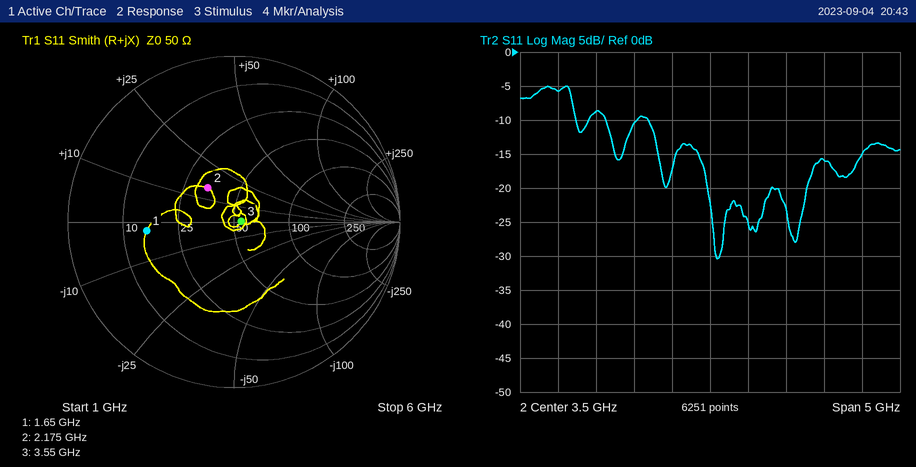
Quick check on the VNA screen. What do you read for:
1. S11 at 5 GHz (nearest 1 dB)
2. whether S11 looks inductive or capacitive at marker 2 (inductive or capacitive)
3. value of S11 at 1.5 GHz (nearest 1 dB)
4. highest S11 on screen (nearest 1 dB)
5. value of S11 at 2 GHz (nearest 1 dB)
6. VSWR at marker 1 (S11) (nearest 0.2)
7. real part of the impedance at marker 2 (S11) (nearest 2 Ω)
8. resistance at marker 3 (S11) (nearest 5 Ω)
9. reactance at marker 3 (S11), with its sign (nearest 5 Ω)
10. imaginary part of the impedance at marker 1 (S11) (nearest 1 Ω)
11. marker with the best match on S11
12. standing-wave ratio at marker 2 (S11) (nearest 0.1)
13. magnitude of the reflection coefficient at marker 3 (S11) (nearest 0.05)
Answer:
-16 dB
inductive
-6 dB
-5 dB
-9 dB
3.2
34 Ω
55 Ω
0 Ω
-2 Ω
marker 3
1.7
0.05
